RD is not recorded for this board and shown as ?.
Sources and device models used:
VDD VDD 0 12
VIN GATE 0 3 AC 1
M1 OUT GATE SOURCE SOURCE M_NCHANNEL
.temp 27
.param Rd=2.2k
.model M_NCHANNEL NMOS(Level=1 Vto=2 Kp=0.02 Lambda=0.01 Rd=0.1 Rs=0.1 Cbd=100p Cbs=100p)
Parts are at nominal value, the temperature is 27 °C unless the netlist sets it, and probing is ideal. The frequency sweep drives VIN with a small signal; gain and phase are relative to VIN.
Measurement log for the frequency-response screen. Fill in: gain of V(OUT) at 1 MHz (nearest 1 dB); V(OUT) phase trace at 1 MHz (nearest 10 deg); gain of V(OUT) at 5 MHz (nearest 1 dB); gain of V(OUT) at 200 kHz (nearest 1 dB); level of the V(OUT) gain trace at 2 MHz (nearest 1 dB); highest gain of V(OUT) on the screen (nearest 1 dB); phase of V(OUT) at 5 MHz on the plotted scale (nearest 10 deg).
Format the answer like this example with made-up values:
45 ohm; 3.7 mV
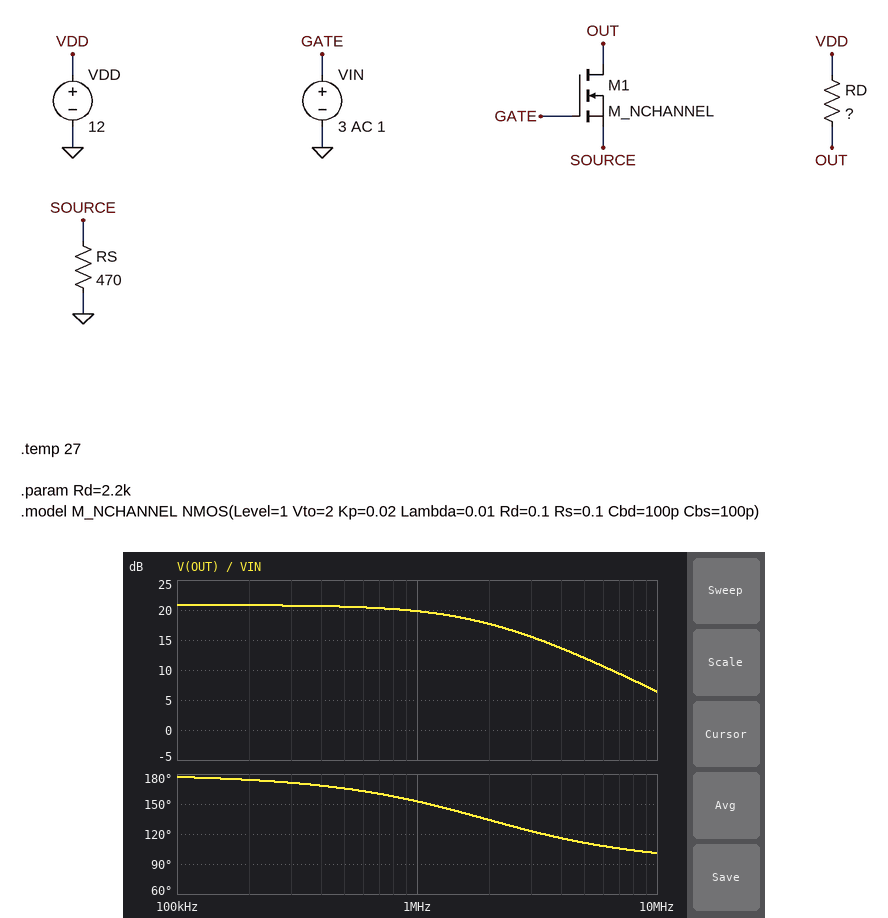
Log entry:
20 dB; 150 deg; 12 dB; 21 dB; 18 dB; 21 dB; 110 deg
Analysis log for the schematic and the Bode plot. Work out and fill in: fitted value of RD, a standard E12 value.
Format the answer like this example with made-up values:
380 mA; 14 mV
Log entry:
6.8 kΩ
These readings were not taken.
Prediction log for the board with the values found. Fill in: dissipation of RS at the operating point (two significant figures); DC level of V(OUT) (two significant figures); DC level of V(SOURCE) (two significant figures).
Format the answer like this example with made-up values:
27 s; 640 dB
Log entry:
860 µW; 2.8 V; 640 mV
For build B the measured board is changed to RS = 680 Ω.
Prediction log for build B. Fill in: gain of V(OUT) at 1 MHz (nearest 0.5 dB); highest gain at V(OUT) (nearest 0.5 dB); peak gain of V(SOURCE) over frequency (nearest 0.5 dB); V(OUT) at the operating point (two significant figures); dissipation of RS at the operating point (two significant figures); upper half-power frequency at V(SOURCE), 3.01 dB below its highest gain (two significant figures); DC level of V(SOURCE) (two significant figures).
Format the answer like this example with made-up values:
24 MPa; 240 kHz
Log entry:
17.5 dB; 18.0 dB; -2.0 dB; 5.1 V; 700 µW; 3.0 MHz; 690 mV
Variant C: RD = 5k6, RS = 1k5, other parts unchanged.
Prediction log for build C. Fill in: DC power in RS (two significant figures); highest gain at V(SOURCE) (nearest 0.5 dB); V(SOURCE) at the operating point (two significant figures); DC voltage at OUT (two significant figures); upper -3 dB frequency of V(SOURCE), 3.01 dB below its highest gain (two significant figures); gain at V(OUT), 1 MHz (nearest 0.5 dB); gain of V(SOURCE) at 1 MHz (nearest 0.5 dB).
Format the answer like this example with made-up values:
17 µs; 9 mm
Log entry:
410 µW; -1.0 dB; 780 mV; 9.1 V; 6.2 MHz; 10.0 dB; -1.5 dB
